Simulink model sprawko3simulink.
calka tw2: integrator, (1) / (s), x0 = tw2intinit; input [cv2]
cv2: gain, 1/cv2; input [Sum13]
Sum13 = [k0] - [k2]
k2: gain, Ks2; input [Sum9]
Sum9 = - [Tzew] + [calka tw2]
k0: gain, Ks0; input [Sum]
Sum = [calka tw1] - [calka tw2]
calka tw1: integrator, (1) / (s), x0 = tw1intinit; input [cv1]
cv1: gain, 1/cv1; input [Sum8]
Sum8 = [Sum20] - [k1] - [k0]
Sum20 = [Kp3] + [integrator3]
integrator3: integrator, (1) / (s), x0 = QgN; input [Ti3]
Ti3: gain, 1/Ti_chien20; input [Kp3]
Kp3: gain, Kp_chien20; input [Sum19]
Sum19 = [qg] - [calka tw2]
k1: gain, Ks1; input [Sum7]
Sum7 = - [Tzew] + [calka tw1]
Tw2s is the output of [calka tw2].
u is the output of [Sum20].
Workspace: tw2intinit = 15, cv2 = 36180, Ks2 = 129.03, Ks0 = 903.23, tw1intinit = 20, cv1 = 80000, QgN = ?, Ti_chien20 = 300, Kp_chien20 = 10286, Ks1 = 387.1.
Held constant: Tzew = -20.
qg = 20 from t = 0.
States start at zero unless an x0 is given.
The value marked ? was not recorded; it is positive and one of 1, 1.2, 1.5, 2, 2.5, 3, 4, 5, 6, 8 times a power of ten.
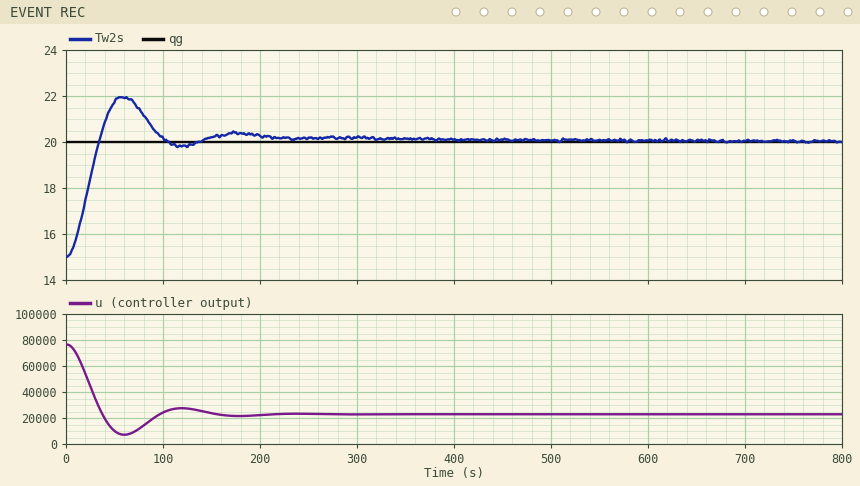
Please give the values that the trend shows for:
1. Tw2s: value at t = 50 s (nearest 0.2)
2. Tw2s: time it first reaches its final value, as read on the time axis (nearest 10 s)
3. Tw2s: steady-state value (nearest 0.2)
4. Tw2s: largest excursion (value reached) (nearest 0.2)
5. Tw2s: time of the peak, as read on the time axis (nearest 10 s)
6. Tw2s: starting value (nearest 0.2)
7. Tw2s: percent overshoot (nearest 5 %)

21.8
30 s
20.0
22.0
60 s
15.0
40 %
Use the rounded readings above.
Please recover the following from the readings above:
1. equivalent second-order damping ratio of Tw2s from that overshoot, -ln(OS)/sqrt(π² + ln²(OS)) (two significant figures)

0.28
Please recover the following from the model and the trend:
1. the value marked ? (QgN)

25000
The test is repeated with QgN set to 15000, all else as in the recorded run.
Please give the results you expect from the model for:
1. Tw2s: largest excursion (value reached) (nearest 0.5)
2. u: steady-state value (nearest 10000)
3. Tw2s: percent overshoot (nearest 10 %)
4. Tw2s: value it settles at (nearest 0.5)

21.0
20000
20 %
20.0
